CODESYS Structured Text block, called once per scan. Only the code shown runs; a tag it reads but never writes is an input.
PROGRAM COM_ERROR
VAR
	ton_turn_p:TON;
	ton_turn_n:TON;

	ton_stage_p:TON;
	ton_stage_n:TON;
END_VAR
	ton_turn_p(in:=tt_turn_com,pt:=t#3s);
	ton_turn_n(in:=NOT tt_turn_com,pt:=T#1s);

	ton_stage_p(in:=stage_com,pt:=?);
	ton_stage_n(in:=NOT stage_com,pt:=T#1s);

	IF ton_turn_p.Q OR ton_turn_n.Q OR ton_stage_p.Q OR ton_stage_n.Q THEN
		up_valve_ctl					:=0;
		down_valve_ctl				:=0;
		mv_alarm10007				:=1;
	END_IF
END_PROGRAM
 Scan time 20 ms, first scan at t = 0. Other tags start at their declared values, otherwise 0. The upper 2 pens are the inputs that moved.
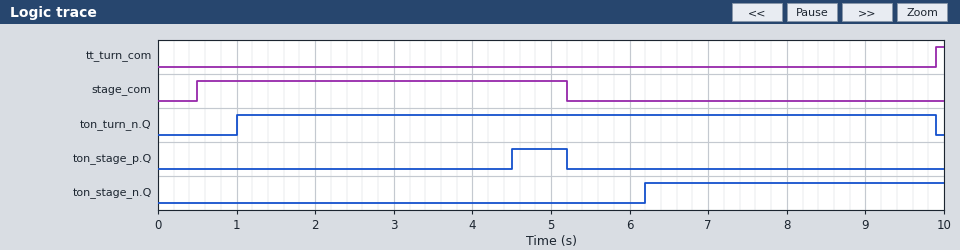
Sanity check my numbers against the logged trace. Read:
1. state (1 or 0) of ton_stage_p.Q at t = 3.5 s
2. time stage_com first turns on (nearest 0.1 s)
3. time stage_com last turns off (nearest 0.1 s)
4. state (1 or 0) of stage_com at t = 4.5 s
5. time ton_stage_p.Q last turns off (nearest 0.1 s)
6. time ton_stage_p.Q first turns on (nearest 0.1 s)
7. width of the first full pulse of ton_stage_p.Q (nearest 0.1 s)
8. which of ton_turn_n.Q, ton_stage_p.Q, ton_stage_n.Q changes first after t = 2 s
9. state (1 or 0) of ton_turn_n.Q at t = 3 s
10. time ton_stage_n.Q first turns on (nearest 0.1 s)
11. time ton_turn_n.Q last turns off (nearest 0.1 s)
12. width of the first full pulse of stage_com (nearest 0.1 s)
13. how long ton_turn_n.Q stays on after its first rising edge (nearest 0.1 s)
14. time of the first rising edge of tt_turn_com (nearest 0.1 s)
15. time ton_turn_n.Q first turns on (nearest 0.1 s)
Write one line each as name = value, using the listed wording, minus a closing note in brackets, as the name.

state (1 or 0) of ton_stage_p.Q at t = 3.5 s = 0
time stage_com first turns on = 0.5 s
time stage_com last turns off = 5.2 s
state (1 or 0) of stage_com at t = 4.5 s = 1
time ton_stage_p.Q last turns off = 5.2 s
time ton_stage_p.Q first turns on = 4.5 s
width of the first full pulse of ton_stage_p.Q = 0.7 s
which of ton_turn_n.Q, ton_stage_p.Q, ton_stage_n.Q changes first after t = 2 s = ton_stage_p.Q
state (1 or 0) of ton_turn_n.Q at t = 3 s = 1
time ton_stage_n.Q first turns on = 6.2 s
time ton_turn_n.Q last turns off = 9.9 s
width of the first full pulse of stage_com = 4.7 s
how long ton_turn_n.Q stays on after its first rising edge = 8.9 s
time of the first rising edge of tt_turn_com = 9.9 s
time ton_turn_n.Q first turns on = 1.0 s
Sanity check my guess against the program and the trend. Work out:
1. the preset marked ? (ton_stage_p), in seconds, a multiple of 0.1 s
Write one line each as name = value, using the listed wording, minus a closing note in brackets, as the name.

the preset marked ? (ton_stage_p), in seconds, a multiple of 0.1 s = 4.0 s
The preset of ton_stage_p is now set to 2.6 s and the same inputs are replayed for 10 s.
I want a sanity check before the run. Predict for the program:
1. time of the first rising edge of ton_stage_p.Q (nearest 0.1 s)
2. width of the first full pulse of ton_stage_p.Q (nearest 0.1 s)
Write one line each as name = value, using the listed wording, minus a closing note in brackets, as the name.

time of the first rising edge of ton_stage_p.Q = 3.1 s
width of the first full pulse of ton_stage_p.Q = 2.1 s
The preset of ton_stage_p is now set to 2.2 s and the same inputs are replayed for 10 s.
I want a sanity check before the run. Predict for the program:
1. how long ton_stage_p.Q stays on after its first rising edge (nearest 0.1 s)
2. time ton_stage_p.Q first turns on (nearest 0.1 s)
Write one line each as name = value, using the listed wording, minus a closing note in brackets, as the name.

how long ton_stage_p.Q stays on after its first rising edge = 2.5 s
time ton_stage_p.Q first turns on = 2.7 s
